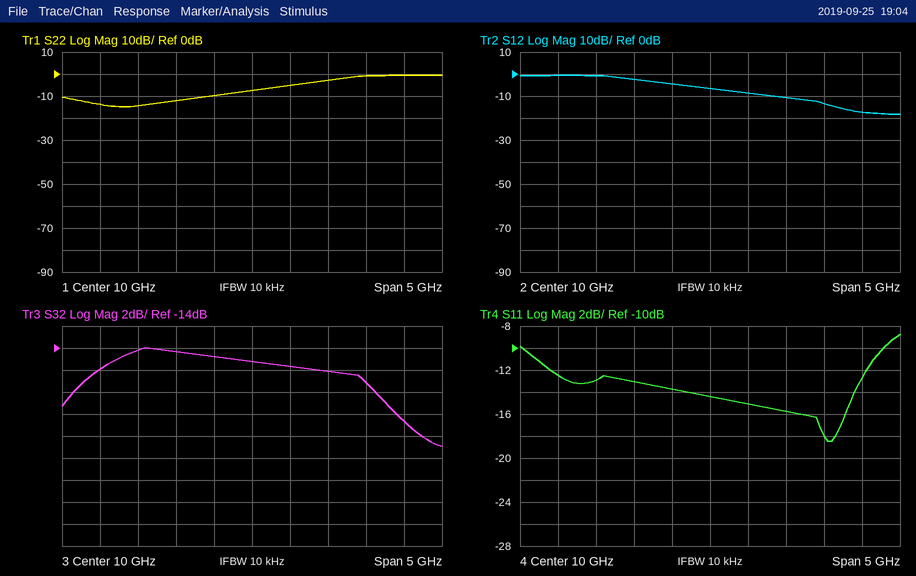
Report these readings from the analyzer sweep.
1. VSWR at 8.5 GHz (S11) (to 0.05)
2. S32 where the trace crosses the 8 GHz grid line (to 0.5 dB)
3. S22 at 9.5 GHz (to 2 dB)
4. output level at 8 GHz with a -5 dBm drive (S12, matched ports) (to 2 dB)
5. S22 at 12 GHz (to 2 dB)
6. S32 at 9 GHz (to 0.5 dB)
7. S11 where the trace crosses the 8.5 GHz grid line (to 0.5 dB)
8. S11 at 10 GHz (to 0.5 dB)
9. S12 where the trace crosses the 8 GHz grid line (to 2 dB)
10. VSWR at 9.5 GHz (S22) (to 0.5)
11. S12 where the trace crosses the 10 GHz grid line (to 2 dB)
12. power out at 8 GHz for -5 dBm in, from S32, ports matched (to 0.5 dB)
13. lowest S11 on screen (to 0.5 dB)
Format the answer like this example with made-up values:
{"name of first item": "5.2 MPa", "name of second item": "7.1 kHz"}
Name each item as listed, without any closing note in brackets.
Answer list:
{"VSWR at 8.5 GHz (S11)": "1.60", "S32 where the trace crosses the 8 GHz grid line": "-16.0 dB", "S22 at 9.5 GHz": "-10 dB", "output level at 8 GHz with a -5 dBm drive (S12, matched ports)": "-6 dBm", "S22 at 12 GHz": "0 dB", "S32 at 9 GHz": "-14.5 dB", "S11 where the trace crosses the 8.5 GHz grid line": "-13.0 dB", "S11 at 10 GHz": "-14.5 dB", "S12 where the trace crosses the 8 GHz grid line": "0 dB", "VSWR at 9.5 GHz (S22)": "2.0", "S12 where the trace crosses the 10 GHz grid line": "-6 dB", "power out at 8 GHz for -5 dBm in, from S32, ports matched": "-21.0 dBm", "lowest S11 on screen": "-18.5 dB"}
